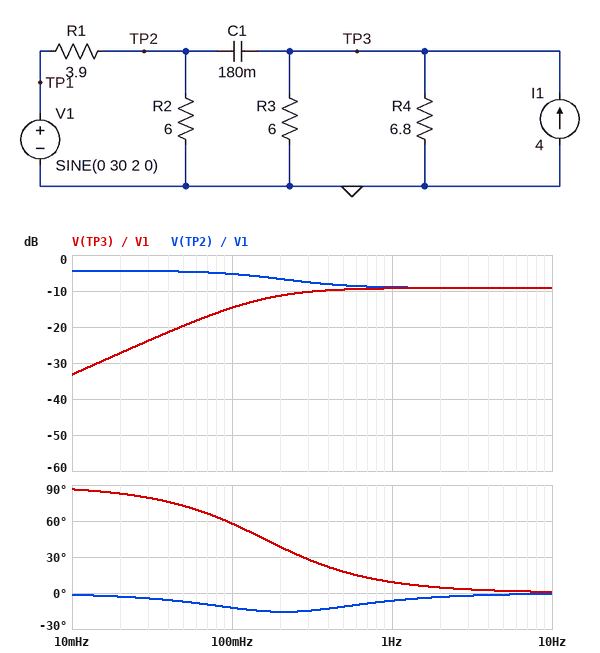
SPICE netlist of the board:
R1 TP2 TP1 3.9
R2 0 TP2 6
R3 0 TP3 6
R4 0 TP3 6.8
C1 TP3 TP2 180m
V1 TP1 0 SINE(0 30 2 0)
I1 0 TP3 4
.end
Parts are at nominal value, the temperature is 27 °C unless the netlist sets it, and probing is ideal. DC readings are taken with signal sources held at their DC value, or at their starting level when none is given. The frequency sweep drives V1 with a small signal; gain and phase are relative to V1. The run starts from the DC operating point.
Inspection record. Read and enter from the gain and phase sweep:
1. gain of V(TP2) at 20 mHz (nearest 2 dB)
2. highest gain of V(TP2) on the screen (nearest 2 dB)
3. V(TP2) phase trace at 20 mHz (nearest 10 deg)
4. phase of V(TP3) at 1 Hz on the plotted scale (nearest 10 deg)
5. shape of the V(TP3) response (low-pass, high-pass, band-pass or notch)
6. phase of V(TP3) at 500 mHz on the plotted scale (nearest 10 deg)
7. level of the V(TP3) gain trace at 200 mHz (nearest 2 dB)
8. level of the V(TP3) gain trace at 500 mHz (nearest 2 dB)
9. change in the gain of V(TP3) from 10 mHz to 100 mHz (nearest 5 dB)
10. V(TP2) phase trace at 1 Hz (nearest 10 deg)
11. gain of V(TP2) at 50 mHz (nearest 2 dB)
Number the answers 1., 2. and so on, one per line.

1. -4 dB
2. -4 dB
3. 0 deg
4. 10 deg
5. high-pass
6. 20 deg
7. -12 dB
8. -10 dB
9. 20 dB
10. -10 deg
11. -4 dB
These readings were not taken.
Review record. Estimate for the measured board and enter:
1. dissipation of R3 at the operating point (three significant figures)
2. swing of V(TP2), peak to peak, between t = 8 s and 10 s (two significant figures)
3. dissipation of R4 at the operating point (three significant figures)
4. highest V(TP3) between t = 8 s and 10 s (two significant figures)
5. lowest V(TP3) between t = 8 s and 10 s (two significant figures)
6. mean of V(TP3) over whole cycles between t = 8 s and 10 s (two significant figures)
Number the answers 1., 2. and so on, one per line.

1. 27.1 W
2. 21 V
3. 23.9 W
4. 23 V
5. 2.3 V
6. 13 V
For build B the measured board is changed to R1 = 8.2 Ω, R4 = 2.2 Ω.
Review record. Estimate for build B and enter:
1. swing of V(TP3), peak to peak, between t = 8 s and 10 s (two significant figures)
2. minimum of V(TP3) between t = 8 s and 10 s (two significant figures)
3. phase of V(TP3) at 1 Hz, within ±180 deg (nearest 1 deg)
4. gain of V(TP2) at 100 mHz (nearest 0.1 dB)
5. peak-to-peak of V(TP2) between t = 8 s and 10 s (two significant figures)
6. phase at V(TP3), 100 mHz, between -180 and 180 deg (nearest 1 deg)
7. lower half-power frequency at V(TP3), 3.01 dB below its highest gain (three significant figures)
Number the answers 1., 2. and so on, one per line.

1. 8.0 V
2. 2.4 V
3. 10 deg
4. -8.6 dB
5. 8.3 V
6. 60 deg
7. 174 mHz
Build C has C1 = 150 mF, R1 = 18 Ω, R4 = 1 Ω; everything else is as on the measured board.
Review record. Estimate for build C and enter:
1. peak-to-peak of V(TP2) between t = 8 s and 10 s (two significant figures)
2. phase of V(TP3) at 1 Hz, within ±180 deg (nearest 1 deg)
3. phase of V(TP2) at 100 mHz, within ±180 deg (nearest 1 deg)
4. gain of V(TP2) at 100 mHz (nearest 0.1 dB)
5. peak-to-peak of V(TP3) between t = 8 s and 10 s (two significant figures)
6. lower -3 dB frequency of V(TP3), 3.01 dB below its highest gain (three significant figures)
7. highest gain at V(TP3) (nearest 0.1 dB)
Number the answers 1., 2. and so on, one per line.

1. 2.8 V
2. 11 deg
3. -22 deg
4. -13.0 dB
5. 2.4 V
6. 198 mHz
7. -28.0 dB
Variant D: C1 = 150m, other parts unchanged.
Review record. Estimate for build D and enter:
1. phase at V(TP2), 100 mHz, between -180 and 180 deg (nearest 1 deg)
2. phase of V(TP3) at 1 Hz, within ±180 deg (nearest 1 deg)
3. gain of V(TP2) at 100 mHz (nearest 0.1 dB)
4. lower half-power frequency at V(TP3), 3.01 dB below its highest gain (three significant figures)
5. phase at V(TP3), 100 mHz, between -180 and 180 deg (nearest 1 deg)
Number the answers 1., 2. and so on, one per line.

1. -11 deg
2. 11 deg
3. -5.0 dB
4. 191 mHz
5. 62 deg
